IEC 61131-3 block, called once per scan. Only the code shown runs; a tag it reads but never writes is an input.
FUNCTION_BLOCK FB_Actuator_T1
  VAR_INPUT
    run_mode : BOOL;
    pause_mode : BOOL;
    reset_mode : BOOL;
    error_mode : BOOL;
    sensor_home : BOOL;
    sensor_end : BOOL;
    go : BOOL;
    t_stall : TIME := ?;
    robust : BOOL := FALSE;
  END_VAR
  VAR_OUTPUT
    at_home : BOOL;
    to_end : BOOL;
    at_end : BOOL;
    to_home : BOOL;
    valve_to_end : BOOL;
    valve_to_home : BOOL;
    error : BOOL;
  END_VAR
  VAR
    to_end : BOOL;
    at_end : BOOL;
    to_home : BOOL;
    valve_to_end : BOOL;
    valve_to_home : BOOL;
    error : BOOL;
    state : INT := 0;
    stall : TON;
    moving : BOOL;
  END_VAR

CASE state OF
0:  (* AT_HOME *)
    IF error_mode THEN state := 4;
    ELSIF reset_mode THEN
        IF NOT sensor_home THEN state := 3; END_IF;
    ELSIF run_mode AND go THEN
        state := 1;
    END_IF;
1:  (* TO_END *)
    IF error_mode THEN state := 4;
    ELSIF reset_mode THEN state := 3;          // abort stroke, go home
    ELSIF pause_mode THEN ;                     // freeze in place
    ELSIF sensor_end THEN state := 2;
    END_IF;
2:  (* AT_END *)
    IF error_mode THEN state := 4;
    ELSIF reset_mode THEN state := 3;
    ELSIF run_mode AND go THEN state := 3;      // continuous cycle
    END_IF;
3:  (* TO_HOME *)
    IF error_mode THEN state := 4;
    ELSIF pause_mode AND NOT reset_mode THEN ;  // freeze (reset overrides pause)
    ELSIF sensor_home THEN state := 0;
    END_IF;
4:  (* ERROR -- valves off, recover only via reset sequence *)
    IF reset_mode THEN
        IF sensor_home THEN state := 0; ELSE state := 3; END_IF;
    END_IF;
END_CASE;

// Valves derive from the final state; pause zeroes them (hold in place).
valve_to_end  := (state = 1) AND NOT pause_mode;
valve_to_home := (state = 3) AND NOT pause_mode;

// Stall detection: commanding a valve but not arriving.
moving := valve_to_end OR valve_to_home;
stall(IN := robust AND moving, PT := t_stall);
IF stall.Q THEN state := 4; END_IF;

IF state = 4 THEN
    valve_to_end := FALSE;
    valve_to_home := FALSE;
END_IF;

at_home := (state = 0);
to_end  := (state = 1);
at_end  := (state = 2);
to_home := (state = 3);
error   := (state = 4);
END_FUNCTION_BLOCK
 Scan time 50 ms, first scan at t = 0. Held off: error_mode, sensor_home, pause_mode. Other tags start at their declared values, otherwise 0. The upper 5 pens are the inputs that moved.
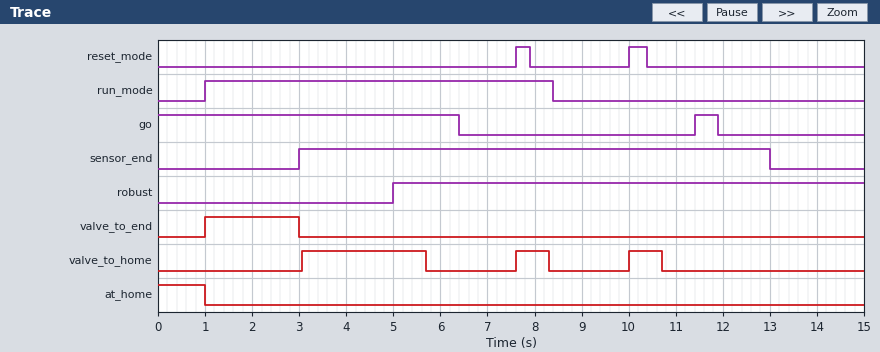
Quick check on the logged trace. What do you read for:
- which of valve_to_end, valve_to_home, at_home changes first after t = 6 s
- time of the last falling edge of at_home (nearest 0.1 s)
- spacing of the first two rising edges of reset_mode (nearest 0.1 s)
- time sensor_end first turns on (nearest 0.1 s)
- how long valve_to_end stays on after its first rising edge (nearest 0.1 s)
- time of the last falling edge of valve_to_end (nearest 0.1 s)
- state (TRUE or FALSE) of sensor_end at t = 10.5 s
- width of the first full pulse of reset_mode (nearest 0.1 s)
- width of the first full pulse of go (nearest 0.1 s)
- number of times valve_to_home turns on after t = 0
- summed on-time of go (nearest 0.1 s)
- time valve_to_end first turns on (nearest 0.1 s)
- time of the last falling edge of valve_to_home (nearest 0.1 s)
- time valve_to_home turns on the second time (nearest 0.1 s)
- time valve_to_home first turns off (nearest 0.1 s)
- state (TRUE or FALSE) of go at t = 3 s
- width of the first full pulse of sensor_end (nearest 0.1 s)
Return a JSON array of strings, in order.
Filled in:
["valve_to_home", "1.0 s", "2.4 s", "3.0 s", "2.0 s", "3.0 s", "TRUE", "0.3 s", "0.5 s", "3", "6.9 s", "1.0 s", "10.7 s", "7.6 s", "5.7 s", "TRUE", "10.0 s"]
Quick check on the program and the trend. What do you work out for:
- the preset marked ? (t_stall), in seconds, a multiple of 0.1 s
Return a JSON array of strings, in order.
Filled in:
["0.7 s"]
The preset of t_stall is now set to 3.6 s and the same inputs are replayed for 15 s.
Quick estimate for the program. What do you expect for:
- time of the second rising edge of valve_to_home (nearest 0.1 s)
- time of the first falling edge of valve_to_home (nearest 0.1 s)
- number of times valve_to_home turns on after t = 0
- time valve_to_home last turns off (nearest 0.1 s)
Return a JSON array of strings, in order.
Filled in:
["10.0 s", "8.6 s", "2", "13.6 s"]
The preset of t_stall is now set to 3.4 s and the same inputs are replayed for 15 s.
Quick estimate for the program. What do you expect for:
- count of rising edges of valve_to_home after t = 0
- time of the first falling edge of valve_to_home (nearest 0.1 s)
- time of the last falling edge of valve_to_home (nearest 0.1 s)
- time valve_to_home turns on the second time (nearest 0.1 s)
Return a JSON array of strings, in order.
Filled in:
["2", "8.4 s", "13.4 s", "10.0 s"]
